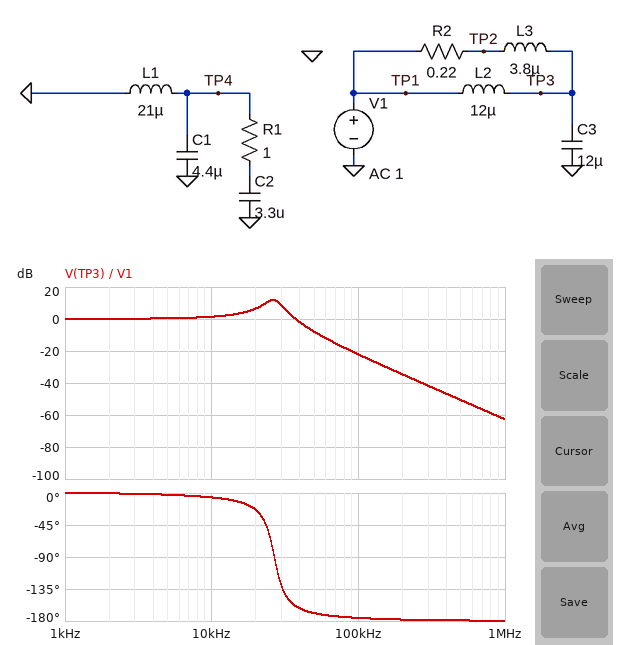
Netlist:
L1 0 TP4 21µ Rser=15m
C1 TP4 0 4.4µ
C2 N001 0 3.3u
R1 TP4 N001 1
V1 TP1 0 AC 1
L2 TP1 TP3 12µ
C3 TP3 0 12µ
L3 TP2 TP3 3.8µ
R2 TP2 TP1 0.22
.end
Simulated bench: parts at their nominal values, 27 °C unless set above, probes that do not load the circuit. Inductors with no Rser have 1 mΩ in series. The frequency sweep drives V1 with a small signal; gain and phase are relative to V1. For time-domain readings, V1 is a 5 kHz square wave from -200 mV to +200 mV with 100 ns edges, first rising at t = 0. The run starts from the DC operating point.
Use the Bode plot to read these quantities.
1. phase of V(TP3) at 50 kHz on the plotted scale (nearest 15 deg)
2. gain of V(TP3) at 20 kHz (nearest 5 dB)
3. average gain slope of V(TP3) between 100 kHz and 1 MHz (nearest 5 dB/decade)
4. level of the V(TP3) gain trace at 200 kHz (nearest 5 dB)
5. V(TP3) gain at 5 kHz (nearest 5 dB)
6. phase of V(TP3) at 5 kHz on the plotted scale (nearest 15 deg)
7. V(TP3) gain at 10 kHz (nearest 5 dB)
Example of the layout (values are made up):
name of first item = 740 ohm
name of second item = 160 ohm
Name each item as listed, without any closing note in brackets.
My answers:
phase of V(TP3) at 50 kHz on the plotted scale = -165 deg
gain of V(TP3) at 20 kHz = 5 dB
average gain slope of V(TP3) between 100 kHz and 1 MHz = -40 dB/decade
level of the V(TP3) gain trace at 200 kHz = -35 dB
V(TP3) gain at 5 kHz = 0 dB
phase of V(TP3) at 5 kHz on the plotted scale = 0 deg
V(TP3) gain at 10 kHz = 0 dB
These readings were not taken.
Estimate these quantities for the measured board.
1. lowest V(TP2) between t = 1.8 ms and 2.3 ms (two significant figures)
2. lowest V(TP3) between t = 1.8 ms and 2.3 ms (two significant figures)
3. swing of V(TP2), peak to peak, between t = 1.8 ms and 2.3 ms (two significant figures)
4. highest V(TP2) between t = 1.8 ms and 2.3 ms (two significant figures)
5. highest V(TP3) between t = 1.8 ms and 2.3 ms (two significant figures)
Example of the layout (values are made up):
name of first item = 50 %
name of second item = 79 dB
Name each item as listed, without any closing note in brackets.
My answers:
lowest V(TP2) between t = 1.8 ms and 2.3 ms = -290 mV
lowest V(TP3) between t = 1.8 ms and 2.3 ms = -500 mV
swing of V(TP2), peak to peak, between t = 1.8 ms and 2.3 ms = 580 mV
highest V(TP2) between t = 1.8 ms and 2.3 ms = 290 mV
highest V(TP3) between t = 1.8 ms and 2.3 ms = 500 mV
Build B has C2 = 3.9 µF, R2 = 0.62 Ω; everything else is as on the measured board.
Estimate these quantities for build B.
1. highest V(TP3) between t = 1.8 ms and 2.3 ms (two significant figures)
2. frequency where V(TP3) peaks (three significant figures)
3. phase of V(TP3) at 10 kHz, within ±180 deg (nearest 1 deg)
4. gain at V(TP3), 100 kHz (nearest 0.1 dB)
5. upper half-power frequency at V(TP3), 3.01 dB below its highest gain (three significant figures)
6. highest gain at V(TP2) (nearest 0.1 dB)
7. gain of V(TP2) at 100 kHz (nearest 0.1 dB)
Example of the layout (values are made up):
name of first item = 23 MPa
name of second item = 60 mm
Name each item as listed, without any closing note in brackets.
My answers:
highest V(TP3) between t = 1.8 ms and 2.3 ms = 380 mV
frequency where V(TP3) peaks = 20.8 kHz
phase of V(TP3) at 10 kHz, within ±180 deg = -15 deg
gain at V(TP3), 100 kHz = -22.4 dB
upper half-power frequency at V(TP3), 3.01 dB below its highest gain = 29.0 kHz
highest gain at V(TP2) = 1.5 dB
gain of V(TP2) at 100 kHz = -0.3 dB
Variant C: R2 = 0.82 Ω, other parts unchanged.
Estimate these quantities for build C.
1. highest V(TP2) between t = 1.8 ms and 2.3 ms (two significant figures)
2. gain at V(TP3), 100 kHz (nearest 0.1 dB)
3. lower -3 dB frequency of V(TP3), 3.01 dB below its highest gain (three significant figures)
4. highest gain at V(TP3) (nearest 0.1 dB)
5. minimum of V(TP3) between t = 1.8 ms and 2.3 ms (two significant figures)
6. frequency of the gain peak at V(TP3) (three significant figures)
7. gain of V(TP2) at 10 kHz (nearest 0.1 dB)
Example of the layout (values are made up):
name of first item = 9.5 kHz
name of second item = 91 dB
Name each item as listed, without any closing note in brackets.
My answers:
highest V(TP2) between t = 1.8 ms and 2.3 ms = 340 mV
gain at V(TP3), 100 kHz = -22.6 dB
lower -3 dB frequency of V(TP3), 3.01 dB below its highest gain = 5.62 kHz
highest gain at V(TP3) = 4.3 dB
minimum of V(TP3) between t = 1.8 ms and 2.3 ms = -370 mV
frequency of the gain peak at V(TP3) = 16.8 kHz
gain of V(TP2) at 10 kHz = 2.1 dB
